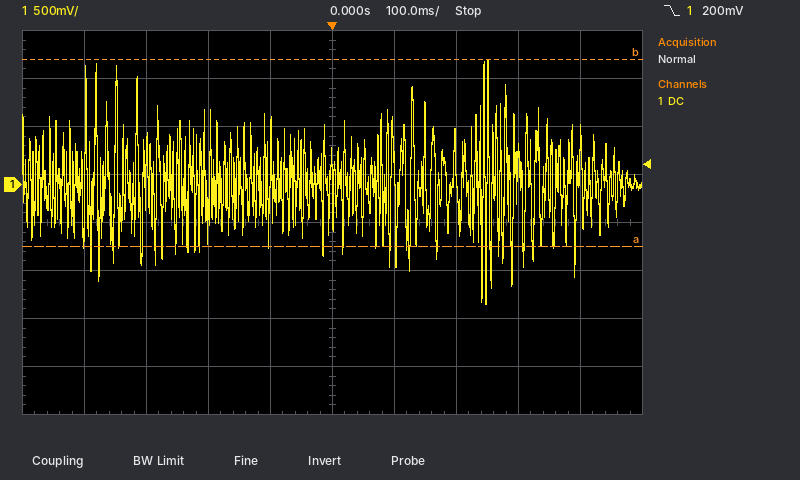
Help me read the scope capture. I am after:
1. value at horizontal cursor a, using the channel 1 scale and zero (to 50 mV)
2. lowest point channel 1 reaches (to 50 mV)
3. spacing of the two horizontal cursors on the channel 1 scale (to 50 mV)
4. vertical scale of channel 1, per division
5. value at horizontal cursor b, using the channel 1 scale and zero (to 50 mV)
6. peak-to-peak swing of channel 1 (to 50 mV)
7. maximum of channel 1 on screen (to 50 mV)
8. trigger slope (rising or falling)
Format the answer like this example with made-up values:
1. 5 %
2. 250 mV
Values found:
1. -650 mV
2. -1.25 V
3. 1.95 V
4. 500 mV
5. 1.30 V
6. 2.55 V
7. 1.30 V
8. falling
